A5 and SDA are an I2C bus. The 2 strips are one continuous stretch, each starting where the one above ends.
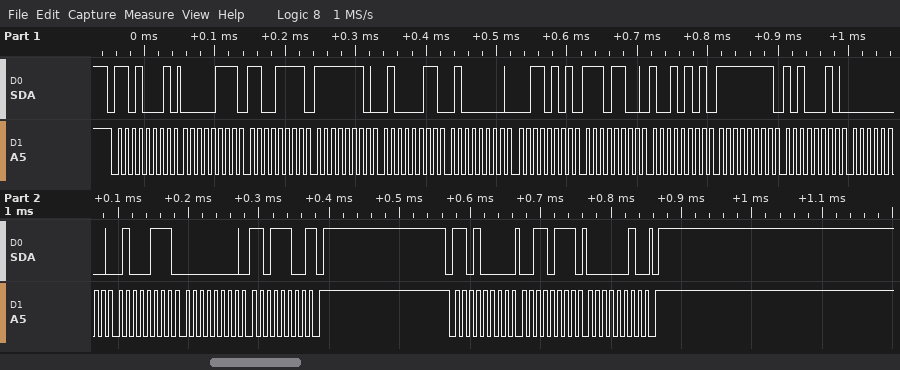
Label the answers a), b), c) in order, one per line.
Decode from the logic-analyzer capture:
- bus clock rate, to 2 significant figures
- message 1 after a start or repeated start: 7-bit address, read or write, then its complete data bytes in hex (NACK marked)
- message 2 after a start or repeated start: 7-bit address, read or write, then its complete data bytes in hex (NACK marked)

a) 100 kHz
b) 0x68 read: 07 CF FE 43 40 35 EC 95 FF A2 00 47 00 DC NACK
c) 0x68 write: 37 02
